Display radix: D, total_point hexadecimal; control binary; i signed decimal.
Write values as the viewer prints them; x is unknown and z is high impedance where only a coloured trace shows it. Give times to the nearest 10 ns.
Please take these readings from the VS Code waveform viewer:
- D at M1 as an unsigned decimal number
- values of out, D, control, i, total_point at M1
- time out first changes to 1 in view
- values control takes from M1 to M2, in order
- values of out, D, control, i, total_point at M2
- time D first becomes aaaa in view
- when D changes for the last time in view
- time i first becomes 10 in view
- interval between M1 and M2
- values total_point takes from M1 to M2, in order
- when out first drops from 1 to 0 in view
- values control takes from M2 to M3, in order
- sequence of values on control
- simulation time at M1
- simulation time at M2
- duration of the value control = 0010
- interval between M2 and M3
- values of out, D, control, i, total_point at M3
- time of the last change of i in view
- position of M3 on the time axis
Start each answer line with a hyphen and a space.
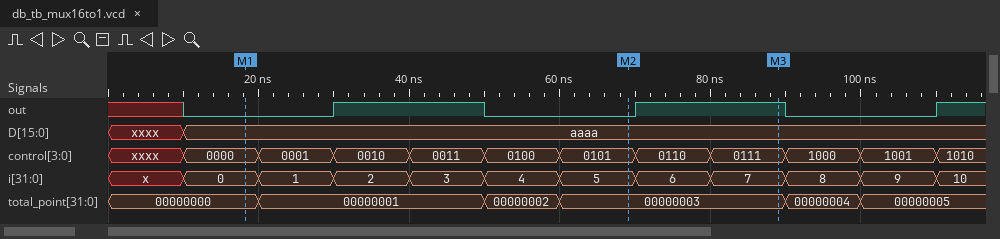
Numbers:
- 43690
- out=0, D=aaaa, control=0000, i=0, total_point=00000000
- 30 ns
- 0000, 0001, 0010, 0011, 0100, 0101
- out=0, D=aaaa, control=0101, i=5, total_point=00000003
- 10 ns
- 10 ns
- 110 ns
- 50 ns
- 00000000, 00000001, 00000002, 00000003
- 50 ns
- 0101, 0110, 0111
- xxxx, 0000, 0001, 0010, 0011, 0100, 0101, 0110, 0111, 1000, 1001, 1010
- 20 ns
- 70 ns
- 10 ns
- 20 ns
- out=1, D=aaaa, control=0111, i=7, total_point=00000003
- 110 ns
- 90 ns
